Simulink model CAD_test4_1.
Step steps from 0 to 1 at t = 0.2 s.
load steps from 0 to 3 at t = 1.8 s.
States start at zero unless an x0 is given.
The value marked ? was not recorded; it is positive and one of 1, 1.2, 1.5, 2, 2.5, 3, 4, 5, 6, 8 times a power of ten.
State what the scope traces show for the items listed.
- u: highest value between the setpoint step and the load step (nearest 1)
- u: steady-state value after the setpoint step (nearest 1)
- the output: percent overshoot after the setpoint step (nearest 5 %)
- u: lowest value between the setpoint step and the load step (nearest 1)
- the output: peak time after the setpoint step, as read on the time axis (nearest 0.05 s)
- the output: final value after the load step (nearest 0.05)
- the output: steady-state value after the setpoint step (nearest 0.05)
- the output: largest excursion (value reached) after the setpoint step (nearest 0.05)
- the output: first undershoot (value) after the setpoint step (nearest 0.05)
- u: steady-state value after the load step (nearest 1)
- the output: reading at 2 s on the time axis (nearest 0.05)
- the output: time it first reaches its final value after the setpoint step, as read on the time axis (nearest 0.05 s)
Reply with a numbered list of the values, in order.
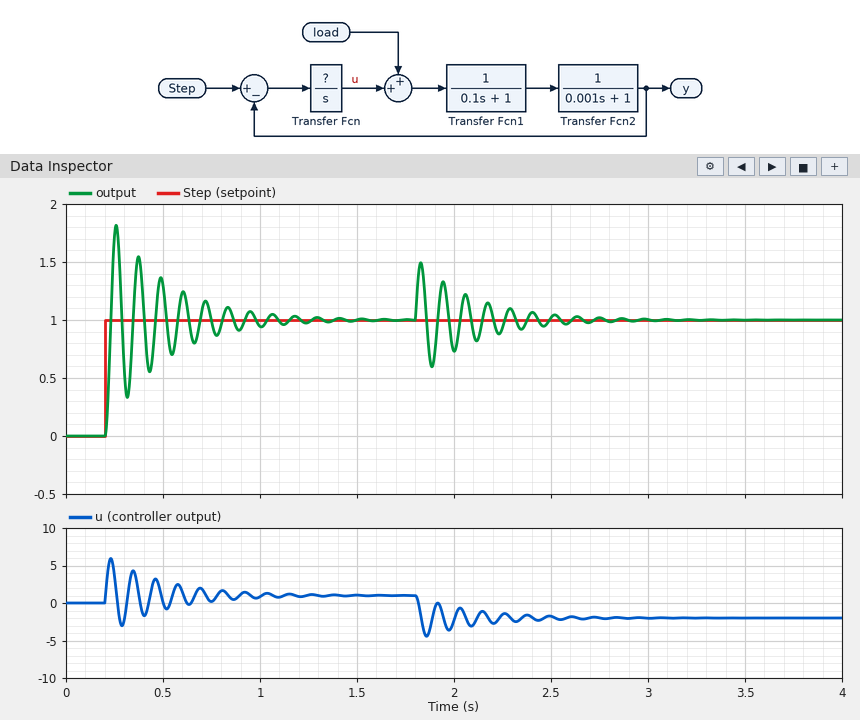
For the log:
1. 6
2. 1
3. 80 %
4. -3
5. 0.25 s
6. 1.00
7. 1.00
8. 1.80
9. 0.35
10. -2
11. 0.75
12. 0.25 s
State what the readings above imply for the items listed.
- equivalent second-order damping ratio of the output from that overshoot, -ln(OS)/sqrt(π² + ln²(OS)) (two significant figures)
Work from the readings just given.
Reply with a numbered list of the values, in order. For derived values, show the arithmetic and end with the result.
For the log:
1. ln(0.8) = -0.223; 0.223 / sqrt(9.870 + 0.050) = 0.071
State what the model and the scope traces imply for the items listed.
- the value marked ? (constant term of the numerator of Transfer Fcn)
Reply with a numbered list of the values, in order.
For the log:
1. 300
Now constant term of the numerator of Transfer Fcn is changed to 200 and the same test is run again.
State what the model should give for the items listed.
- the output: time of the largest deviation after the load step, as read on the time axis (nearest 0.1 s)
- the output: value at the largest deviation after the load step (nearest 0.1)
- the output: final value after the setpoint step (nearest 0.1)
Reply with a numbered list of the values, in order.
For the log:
1. 1.8 s
2. 1.6
3. 1.0
